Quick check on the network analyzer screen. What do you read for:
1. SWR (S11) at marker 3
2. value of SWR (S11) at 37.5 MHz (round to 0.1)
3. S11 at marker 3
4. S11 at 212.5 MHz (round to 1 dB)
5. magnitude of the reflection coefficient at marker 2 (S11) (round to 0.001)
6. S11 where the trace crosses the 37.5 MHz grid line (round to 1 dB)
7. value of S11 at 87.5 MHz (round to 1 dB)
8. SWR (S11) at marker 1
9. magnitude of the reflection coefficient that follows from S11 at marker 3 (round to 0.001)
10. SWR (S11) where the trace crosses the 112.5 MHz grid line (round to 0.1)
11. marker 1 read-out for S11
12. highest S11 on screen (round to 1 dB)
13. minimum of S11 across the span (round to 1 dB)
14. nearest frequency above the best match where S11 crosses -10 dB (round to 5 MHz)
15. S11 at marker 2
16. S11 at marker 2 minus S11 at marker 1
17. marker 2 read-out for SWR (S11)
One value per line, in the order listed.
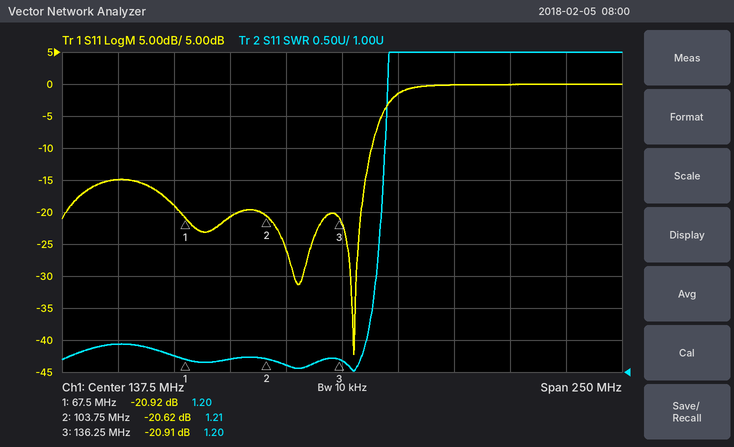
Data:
1.20
1.4
-20.91 dB
0 dB
0.093
-15 dB
-21 dB
1.20
0.090
1.1
-20.92 dB
0 dB
-42 dB
150 MHz
-20.62 dB
0.30 dB
1.21
